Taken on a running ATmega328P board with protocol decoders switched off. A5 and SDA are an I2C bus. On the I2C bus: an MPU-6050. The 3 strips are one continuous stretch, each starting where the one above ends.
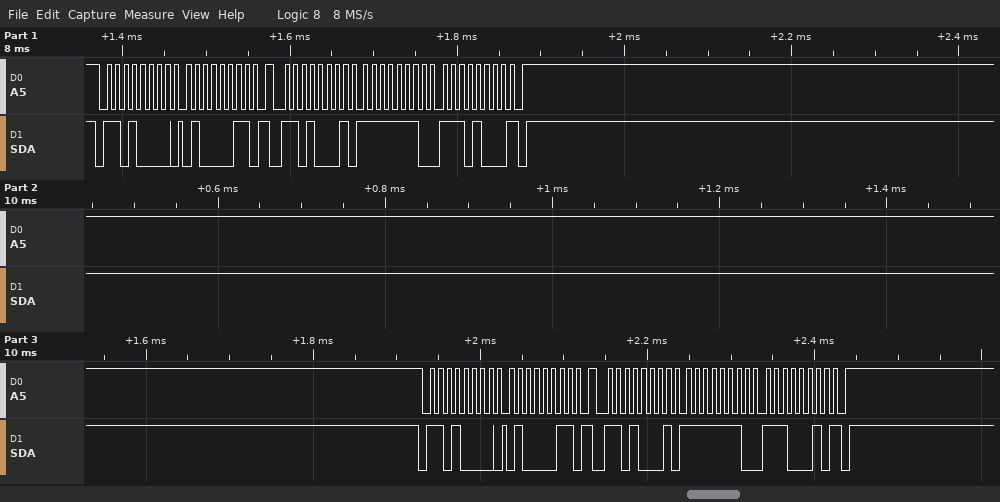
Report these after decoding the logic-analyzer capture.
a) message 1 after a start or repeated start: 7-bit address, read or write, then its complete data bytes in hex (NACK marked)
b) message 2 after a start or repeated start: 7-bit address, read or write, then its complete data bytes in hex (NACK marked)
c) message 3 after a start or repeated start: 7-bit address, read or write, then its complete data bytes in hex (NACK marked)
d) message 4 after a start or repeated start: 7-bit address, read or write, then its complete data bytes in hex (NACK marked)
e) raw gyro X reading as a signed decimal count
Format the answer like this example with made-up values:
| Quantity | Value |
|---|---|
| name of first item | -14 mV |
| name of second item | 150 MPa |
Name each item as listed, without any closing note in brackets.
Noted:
| Quantity | Value |
|---|---|
| message 1 after a start or repeated start: 7-bit address, read or write, then its complete data bytes in hex | 0x68 write: 43 |
| message 2 after a start or repeated start: 7-bit address, read or write, then its complete data bytes in hex | 0x68 read: FE E8 NACK |
| message 3 after a start or repeated start: 7-bit address, read or write, then its complete data bytes in hex | 0x68 write: 43 |
| message 4 after a start or repeated start: 7-bit address, read or write, then its complete data bytes in hex | 0x68 read: FE E2 NACK |
| raw gyro X reading as a signed decimal count | -280 |
